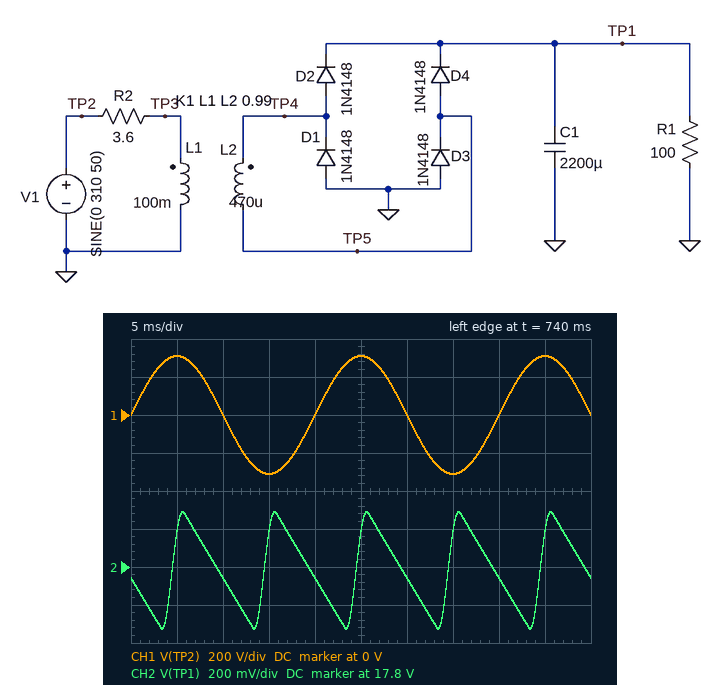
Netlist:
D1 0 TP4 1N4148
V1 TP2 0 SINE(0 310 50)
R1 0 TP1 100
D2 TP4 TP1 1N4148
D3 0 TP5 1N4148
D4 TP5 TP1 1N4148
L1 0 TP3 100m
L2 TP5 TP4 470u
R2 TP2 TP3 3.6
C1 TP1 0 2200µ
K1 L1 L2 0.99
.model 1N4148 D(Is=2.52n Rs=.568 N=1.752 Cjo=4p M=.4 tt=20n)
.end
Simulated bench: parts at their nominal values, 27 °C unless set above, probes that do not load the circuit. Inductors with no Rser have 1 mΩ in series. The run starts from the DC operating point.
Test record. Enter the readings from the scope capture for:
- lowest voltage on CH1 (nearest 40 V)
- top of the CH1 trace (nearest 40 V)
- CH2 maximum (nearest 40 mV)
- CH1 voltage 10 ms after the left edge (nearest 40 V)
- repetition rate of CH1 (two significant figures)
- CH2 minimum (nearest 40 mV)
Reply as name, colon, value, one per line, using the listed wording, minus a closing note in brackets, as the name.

lowest voltage on CH1: -320 V
top of the CH1 trace: 320 V
CH2 maximum: 18.08 V
CH1 voltage 10 ms after the left edge: 0 V
repetition rate of CH1: 50 Hz
CH2 minimum: 17.48 V
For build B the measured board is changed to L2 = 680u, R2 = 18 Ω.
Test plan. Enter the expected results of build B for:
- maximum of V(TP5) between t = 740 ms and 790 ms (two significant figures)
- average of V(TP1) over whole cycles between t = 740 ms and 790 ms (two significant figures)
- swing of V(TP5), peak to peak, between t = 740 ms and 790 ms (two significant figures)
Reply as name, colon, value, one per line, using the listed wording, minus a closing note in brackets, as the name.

maximum of V(TP5) between t = 740 ms and 790 ms: 20 V
average of V(TP1) over whole cycles between t = 740 ms and 790 ms: 19 V
swing of V(TP5), peak to peak, between t = 740 ms and 790 ms: 22 V
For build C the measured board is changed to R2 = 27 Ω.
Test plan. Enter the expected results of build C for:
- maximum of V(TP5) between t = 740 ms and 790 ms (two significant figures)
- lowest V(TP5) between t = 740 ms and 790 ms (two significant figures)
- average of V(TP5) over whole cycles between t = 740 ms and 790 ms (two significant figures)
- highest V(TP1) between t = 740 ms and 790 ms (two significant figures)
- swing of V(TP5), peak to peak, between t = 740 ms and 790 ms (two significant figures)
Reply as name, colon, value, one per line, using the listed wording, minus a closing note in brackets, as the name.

maximum of V(TP5) between t = 740 ms and 790 ms: 15 V
lowest V(TP5) between t = 740 ms and 790 ms: -1.3 V
average of V(TP5) over whole cycles between t = 740 ms and 790 ms: 6.6 V
highest V(TP1) between t = 740 ms and 790 ms: 13 V
swing of V(TP5), peak to peak, between t = 740 ms and 790 ms: 16 V
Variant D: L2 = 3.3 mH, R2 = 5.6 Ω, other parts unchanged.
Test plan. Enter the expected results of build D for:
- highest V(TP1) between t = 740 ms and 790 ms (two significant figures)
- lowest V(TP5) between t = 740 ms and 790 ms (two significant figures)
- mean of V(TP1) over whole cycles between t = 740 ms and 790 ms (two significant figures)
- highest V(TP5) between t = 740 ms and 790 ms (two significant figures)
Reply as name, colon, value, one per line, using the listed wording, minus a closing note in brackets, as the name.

highest V(TP1) between t = 740 ms and 790 ms: 50 V
lowest V(TP5) between t = 740 ms and 790 ms: -2.6 V
mean of V(TP1) over whole cycles between t = 740 ms and 790 ms: 49 V
highest V(TP5) between t = 740 ms and 790 ms: 52 V
